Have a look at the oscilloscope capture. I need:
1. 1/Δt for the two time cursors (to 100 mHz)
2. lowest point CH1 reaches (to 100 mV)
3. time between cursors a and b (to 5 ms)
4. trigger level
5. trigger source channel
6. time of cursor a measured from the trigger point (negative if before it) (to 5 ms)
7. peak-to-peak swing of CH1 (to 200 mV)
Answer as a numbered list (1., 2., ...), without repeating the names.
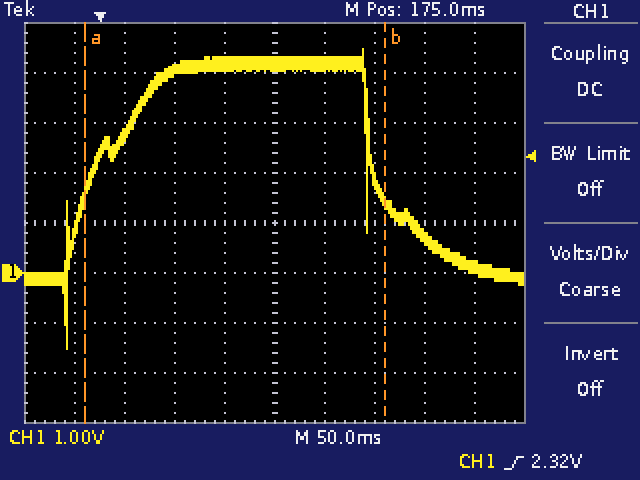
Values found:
1. 3.3 Hz
2. -1.5 V
3. 300 ms
4. 2.32 V
5. CH1
6. -15 ms
7. 6.0 V
